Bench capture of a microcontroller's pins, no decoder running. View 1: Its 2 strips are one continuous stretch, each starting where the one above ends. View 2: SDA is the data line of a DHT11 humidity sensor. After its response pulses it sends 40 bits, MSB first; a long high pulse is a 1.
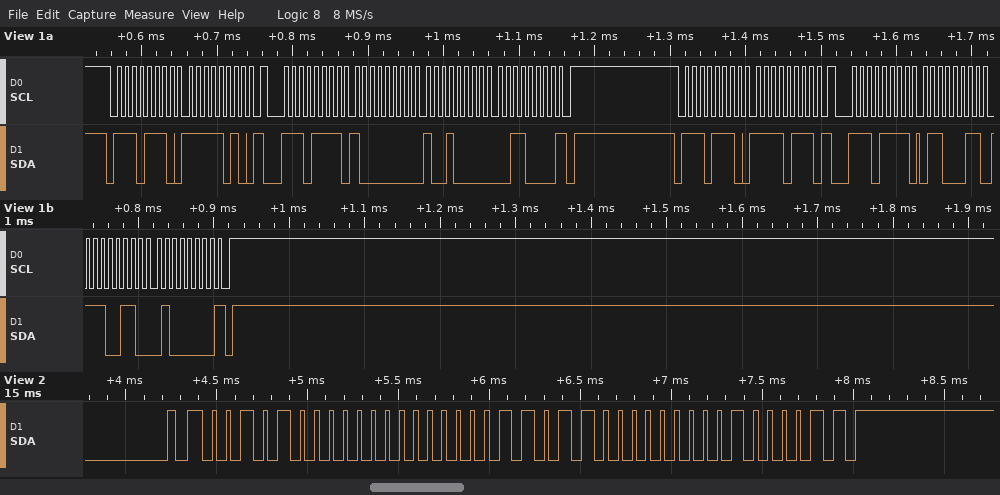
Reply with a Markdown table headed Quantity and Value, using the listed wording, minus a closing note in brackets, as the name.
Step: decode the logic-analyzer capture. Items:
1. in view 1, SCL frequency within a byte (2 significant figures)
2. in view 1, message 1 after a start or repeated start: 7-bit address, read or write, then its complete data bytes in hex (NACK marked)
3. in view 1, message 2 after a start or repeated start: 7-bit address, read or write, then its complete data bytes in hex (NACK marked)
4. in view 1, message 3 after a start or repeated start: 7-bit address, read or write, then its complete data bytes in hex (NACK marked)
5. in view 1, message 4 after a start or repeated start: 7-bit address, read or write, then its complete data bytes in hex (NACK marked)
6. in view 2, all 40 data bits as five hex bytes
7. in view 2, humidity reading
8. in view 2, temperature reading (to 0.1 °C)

| Quantity | Value |
|---|---|
| in view 1, SCL frequency within a byte | 100 kHz |
| in view 1, message 1 after a start or repeated start: 7-bit address, read or write, then its complete data bytes in hex | 0x77 write: FA |
| in view 1, message 2 after a start or repeated start: 7-bit address, read or write, then its complete data bytes in hex | 0x77 read: 80 90 30 NACK |
| in view 1, message 3 after a start or repeated start: 7-bit address, read or write, then its complete data bytes in hex | 0x77 write: F7 |
| in view 1, message 4 after a start or repeated start: 7-bit address, read or write, then its complete data bytes in hex | 0x77 read: 63 E6 40 NACK |
| in view 2, all 40 data bits as five hex bytes | 28 00 1B 00 43 |
| in view 2, humidity reading | 40 % |
| in view 2, temperature reading | 27.0 °C |
